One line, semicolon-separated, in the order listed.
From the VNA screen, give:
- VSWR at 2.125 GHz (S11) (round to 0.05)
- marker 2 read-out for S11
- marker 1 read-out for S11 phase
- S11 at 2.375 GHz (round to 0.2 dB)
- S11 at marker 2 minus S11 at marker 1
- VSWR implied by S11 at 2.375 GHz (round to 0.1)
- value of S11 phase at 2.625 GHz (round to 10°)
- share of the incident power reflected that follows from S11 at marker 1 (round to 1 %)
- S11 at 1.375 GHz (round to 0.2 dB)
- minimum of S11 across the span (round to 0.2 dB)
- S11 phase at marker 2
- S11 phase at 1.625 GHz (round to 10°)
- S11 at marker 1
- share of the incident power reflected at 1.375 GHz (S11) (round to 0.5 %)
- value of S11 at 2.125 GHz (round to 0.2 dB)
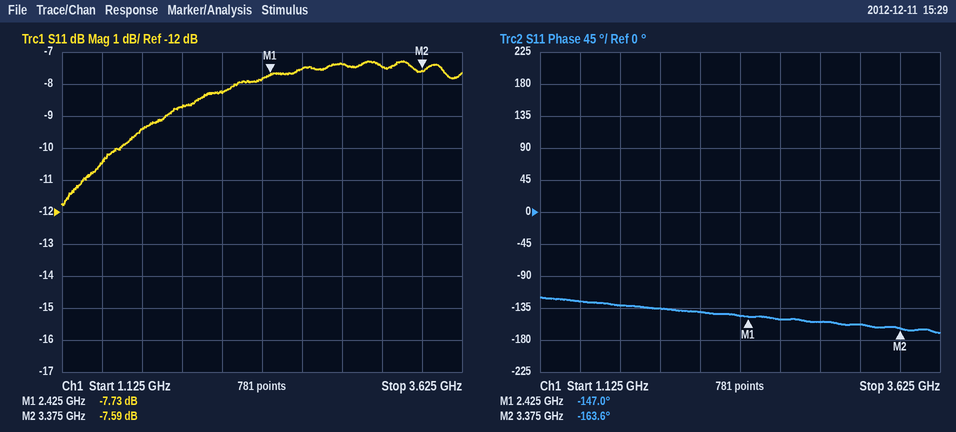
2.25; -7.59 dB; -147.0°; -7.8 dB; 0.14 dB; 2.4; -150°; 17 %; -10.4 dB; -11.8 dB; -163.6°; -130°; -7.73 dB; 9.0 %; -8.2 dB
